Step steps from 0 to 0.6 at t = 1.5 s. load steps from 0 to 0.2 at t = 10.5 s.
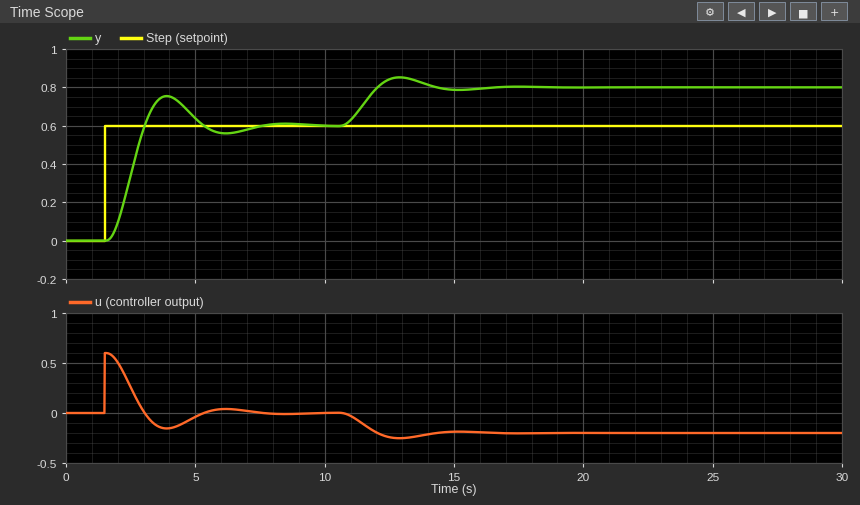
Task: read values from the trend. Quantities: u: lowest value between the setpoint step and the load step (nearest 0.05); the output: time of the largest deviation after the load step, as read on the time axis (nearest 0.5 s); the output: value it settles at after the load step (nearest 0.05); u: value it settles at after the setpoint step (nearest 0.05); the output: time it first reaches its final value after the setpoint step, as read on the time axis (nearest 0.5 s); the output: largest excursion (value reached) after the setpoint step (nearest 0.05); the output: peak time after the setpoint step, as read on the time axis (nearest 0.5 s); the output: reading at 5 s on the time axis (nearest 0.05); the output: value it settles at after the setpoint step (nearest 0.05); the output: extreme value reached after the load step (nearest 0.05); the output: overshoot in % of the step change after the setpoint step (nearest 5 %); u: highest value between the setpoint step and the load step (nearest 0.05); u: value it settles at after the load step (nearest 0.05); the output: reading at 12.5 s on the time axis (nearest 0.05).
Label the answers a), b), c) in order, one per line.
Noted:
a) -0.15
b) 13.0 s
c) 0.80
d) 0.00
e) 3.0 s
f) 0.75
g) 4.0 s
h) 0.65
i) 0.60
j) 0.85
k) 25 %
l) 0.60
m) -0.20
n) 0.85
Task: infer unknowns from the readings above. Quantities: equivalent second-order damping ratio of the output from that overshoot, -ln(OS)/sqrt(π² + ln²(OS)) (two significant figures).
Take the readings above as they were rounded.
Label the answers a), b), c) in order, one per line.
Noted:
a) 0.40
